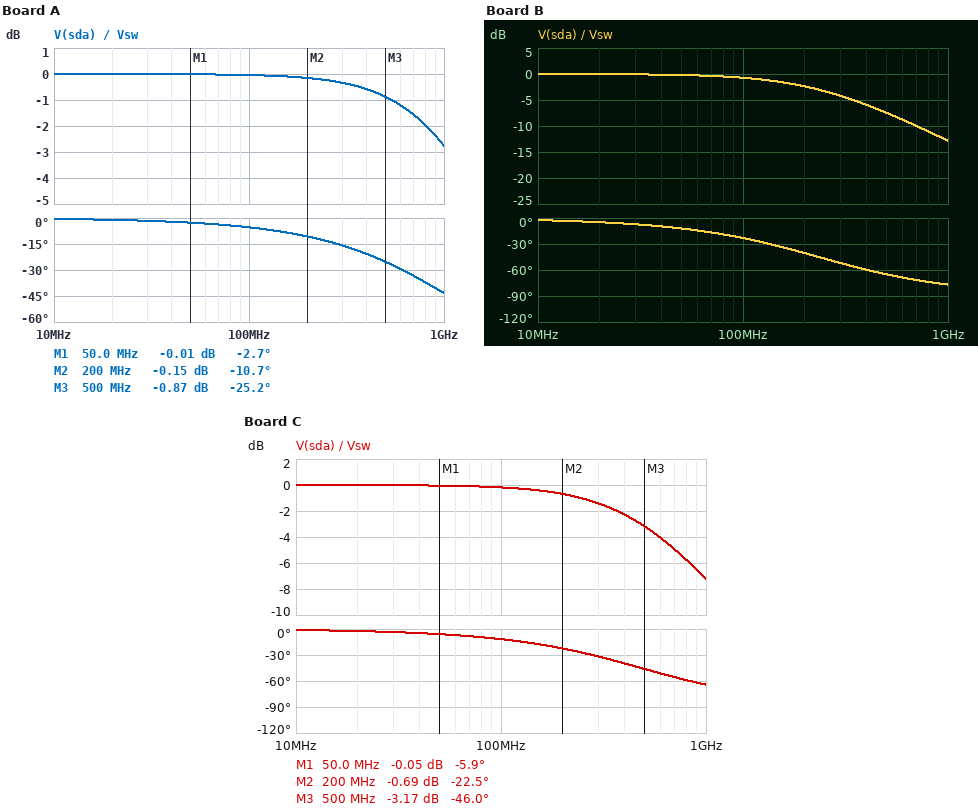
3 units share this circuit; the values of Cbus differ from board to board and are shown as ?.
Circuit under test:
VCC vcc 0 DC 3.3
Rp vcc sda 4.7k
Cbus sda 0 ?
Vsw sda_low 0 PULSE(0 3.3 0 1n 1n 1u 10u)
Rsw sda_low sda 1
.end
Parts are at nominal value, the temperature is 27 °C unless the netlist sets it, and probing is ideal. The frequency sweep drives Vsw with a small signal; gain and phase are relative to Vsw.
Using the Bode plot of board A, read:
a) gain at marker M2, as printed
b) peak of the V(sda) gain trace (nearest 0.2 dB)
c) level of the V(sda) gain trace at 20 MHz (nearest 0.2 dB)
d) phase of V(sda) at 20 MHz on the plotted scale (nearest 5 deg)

-0.15 dB
0 dB
0 dB
0 deg
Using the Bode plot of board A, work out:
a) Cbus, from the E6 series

150 pF
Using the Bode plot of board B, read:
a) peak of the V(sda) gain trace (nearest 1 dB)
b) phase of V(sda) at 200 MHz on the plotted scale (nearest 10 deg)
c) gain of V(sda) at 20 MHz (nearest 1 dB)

0 dB
-40 deg
0 dB
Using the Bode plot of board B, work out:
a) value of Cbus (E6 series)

680 pF
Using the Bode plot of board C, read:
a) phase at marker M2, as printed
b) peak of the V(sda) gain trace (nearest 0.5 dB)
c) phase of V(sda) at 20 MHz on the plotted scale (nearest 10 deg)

-22.5 deg
0 dB
0 deg
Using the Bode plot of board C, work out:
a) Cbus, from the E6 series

330 pF
